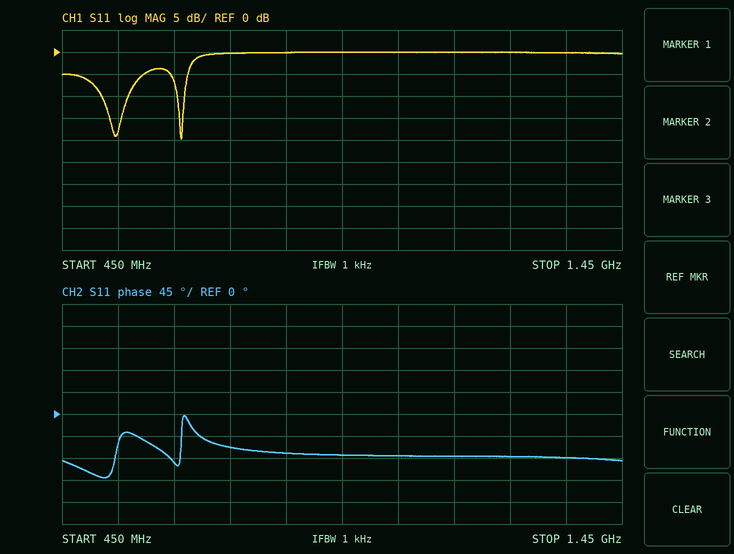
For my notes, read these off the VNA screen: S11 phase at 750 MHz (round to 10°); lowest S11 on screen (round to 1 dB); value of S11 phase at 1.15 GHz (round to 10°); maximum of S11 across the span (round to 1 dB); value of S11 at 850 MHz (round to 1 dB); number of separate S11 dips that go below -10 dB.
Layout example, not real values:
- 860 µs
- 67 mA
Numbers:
- -70°
- -20 dB
- -90°
- 0 dB
- 0 dB
- 2
